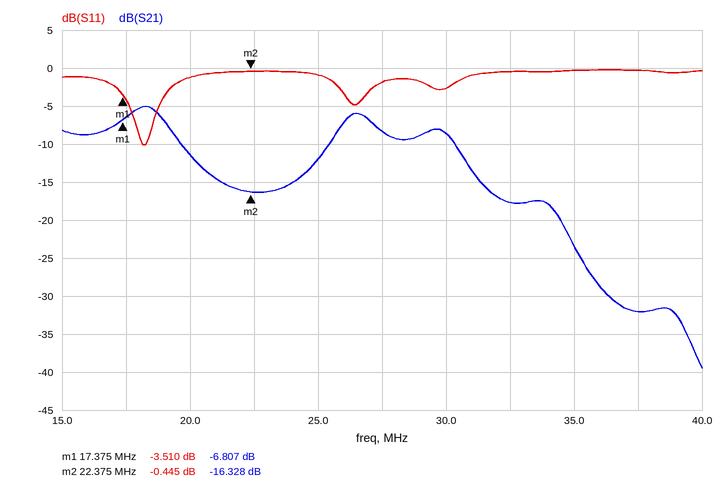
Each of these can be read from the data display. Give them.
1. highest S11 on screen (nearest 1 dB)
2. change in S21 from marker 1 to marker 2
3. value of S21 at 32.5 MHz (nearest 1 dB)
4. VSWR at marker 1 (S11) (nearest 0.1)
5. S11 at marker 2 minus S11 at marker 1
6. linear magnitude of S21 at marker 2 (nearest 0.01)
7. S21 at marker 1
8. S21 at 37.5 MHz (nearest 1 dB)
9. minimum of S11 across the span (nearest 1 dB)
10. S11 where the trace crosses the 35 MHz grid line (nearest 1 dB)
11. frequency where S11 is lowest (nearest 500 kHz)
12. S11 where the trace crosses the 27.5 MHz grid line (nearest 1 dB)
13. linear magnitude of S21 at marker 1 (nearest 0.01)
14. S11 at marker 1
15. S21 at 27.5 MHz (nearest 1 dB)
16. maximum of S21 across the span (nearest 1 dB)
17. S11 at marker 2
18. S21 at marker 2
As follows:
0 dB
-9.521 dB
-18 dB
5.0
3.065 dB
0.15
-6.807 dB
-32 dB
-10 dB
0 dB
18.0 MHz
-2 dB
0.46
-3.510 dB
-8 dB
-5 dB
-0.445 dB
-16.328 dB
